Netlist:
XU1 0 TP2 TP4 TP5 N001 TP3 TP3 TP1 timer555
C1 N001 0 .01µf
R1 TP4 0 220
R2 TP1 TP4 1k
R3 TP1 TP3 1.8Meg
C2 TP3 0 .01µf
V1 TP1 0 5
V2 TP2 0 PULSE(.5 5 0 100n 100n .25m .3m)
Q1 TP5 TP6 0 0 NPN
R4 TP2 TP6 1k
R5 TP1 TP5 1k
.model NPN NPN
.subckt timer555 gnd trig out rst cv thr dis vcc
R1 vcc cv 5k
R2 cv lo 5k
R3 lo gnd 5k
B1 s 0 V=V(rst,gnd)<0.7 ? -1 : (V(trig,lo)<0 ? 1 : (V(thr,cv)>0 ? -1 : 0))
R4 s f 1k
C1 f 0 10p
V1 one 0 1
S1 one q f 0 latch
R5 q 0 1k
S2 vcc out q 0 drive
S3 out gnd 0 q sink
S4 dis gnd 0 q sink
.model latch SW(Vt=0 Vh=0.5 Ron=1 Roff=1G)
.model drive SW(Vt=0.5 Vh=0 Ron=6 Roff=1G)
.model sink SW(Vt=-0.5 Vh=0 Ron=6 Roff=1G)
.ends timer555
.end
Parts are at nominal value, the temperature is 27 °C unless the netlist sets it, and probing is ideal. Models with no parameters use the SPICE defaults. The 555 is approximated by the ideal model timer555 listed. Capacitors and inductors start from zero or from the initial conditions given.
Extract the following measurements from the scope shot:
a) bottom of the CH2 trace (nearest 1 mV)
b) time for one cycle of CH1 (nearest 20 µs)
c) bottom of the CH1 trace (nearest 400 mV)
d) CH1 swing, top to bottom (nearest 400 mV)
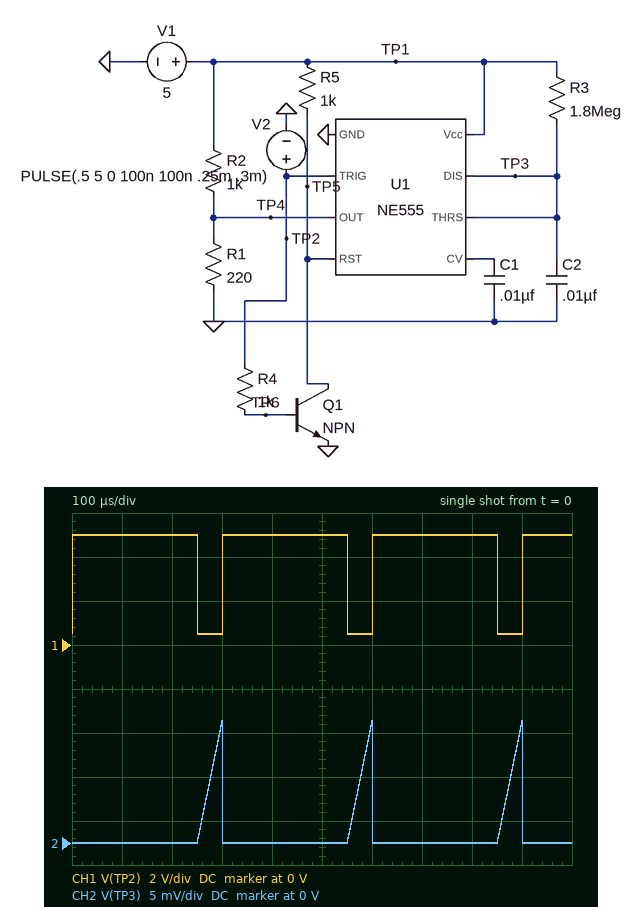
0 V
300 µs
400 mV
4.4 V
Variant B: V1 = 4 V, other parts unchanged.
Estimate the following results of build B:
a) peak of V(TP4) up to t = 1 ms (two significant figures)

3.9 V
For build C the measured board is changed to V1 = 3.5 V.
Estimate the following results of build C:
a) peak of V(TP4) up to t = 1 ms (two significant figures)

3.4 V
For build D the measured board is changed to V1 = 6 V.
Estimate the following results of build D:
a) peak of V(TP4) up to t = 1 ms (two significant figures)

5.8 V
